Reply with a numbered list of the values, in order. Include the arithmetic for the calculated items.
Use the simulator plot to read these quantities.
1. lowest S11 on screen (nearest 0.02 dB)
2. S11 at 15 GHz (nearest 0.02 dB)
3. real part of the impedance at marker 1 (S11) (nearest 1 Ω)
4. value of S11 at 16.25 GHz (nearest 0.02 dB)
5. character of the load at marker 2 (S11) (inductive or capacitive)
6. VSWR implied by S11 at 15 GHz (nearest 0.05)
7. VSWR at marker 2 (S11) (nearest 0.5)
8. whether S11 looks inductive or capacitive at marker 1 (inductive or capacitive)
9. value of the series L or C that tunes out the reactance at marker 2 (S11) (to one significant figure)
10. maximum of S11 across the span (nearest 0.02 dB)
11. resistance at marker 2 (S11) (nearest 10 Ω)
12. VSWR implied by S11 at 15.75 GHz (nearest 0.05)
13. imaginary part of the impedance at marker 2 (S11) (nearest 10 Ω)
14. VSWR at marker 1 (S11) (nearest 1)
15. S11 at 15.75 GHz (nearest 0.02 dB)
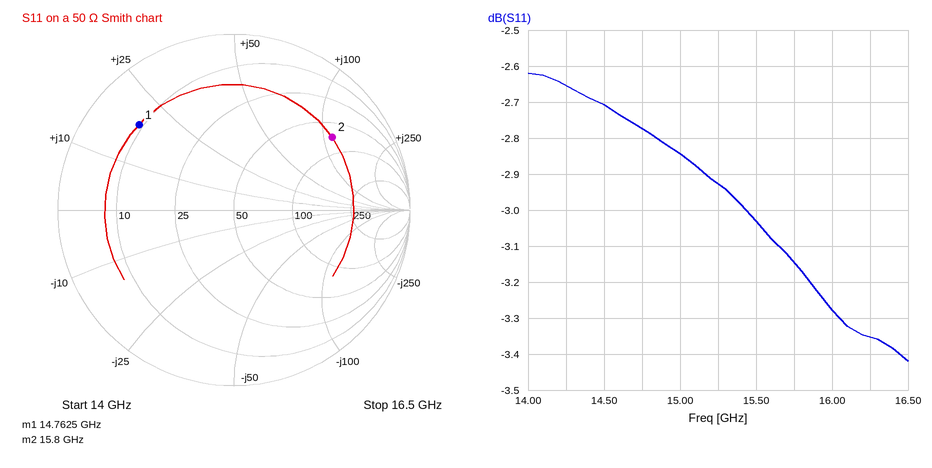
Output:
1. -3.42 dB
2. -2.84 dB
3. 9 Ω
4. -3.36 dB
5. inductive
6. |Γ| = 10^(-2.84/20) = 0.7211; VSWR = (1 + 0.7211)/(1 − 0.7211) ≈ 6.17, so 6.15 to the nearest 0.05
7. 5.5
8. inductive
9. C = 1/(2π × 15.8 GHz × 110 Ω) ≈ 91.6 fF, so 90 fF to one significant figure
10. -2.62 dB
11. 70 Ω
12. |Γ| = 10^(-3.14/20) = 0.6966; VSWR = (1 + 0.6966)/(1 − 0.6966) ≈ 5.59, so 5.60 to the nearest 0.05
13. +110 Ω
14. 6
15. -3.14 dB
